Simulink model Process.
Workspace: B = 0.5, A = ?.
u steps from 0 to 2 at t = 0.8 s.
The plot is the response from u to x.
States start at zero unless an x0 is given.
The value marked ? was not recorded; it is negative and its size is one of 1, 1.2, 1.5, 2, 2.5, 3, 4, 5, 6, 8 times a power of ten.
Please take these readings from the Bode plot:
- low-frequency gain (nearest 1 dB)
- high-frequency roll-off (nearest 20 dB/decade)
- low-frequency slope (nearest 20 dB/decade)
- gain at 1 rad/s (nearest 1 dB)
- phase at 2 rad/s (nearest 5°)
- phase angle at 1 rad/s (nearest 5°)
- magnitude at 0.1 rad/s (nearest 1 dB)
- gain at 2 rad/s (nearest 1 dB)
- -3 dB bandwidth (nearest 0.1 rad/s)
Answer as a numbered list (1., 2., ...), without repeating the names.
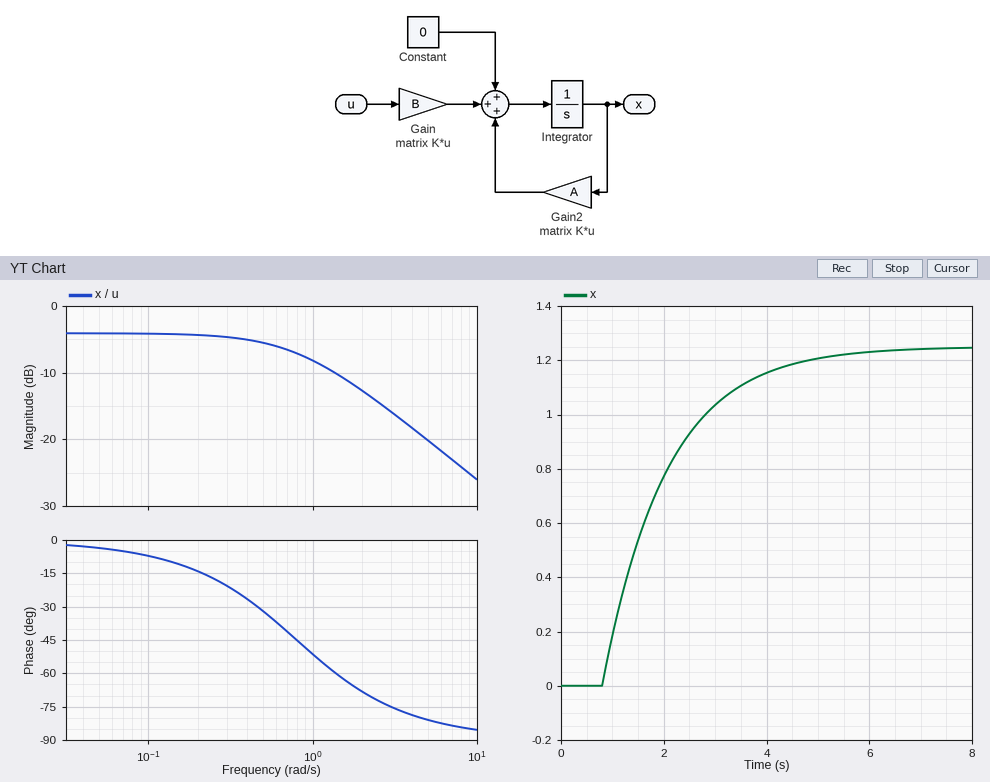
1. -4 dB
2. -20 dB/decade
3. 0 dB/decade
4. -8 dB
5. -70°
6. -50°
7. -4 dB
8. -13 dB
9. 0.8 rad/s
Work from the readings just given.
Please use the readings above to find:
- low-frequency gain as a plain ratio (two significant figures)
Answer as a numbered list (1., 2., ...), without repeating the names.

1. 0.63
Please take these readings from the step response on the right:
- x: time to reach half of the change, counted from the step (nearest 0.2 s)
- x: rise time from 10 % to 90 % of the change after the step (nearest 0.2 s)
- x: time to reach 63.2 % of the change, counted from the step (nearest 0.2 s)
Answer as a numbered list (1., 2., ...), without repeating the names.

1. 0.8 s
2. 2.8 s
3. 1.2 s
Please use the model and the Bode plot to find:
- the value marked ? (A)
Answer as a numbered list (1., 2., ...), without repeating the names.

1. -0.8
